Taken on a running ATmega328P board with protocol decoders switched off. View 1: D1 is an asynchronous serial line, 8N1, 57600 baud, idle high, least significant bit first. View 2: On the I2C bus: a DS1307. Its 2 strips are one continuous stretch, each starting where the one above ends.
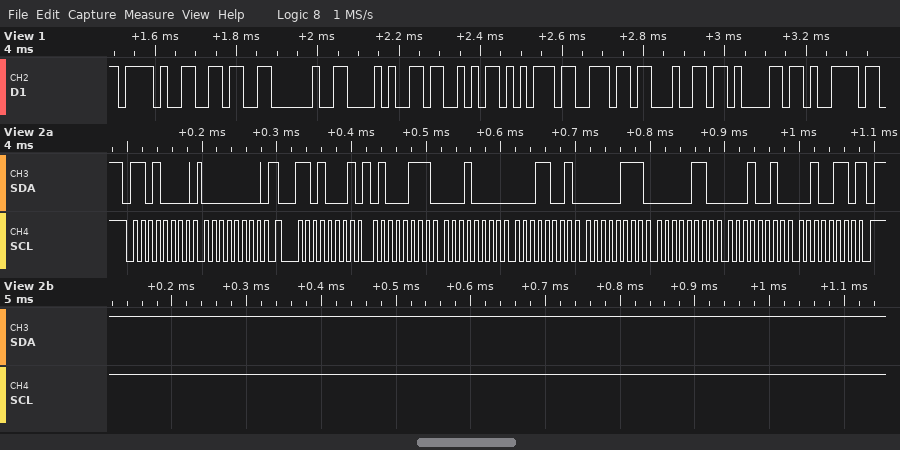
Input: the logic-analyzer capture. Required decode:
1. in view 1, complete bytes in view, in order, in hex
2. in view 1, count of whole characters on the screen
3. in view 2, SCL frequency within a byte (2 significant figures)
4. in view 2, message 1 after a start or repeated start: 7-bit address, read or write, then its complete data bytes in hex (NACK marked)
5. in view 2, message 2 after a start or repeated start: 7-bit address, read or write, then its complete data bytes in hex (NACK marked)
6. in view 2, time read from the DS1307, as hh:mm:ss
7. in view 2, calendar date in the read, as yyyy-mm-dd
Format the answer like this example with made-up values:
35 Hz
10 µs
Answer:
2F 36 20 28 53 75 6E 64 61 79
10
100 kHz
0x68 write: 00
0x68 read: 47 10 19 07 06 12 26 NACK
19:10:47
2026-12-06
